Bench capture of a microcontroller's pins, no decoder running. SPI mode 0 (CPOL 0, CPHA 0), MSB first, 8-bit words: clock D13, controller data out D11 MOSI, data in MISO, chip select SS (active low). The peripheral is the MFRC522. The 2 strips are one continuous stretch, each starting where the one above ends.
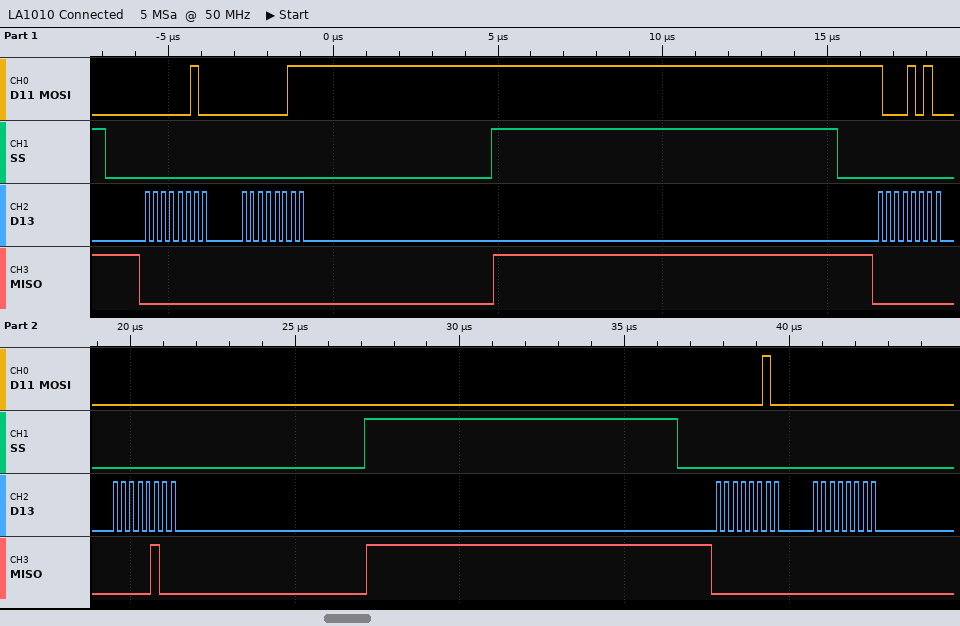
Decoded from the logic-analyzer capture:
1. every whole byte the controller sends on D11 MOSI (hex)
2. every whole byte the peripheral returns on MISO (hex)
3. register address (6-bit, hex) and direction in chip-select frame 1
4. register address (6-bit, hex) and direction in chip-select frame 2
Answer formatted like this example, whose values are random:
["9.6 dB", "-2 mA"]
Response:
["02 03 8A 00 02 00", "00 00 00 04 00 00", "0x01 write", "0x05 read"]
